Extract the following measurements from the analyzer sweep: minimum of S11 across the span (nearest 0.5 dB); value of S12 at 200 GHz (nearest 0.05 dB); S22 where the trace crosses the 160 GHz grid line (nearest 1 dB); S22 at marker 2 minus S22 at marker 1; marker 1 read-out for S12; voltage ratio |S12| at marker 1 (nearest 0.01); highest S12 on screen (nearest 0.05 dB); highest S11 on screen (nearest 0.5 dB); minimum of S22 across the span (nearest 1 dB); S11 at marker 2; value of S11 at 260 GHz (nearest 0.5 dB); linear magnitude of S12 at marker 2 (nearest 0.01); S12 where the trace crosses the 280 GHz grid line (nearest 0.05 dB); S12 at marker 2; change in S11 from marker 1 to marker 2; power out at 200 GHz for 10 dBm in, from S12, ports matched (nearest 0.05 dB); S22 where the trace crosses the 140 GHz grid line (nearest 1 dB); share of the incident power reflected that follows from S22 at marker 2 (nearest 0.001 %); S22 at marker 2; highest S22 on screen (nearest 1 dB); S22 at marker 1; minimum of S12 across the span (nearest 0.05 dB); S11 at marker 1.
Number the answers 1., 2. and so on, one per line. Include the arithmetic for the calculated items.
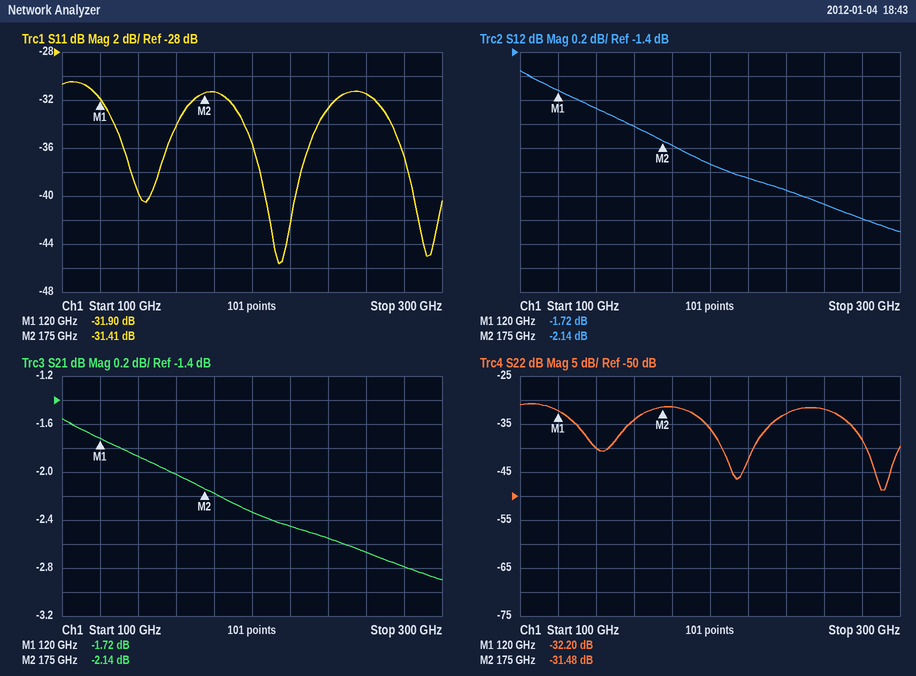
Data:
1. -45.5 dB
2. -2.35 dB
3. -34 dB
4. -31.48 − (-32.2) = 0.72 dB
5. -1.72 dB
6. 10^(-1.72/20) ≈ 0.82
7. -1.55 dB
8. -30.5 dB
9. -49 dB
10. -31.41 dB
11. -31.5 dB
12. 10^(-2.14/20) ≈ 0.78
13. -2.80 dB
14. -2.14 dB
15. -31.41 − (-31.9) = 0.49 dB
16. 10 dBm + (-2.35 dB) = 7.65 dBm
17. -40 dB
18. 10^(-31.48/10) ≈ 0.071 %
19. -31.48 dB
20. -31 dB
21. -32.20 dB
22. -2.90 dB
23. -31.90 dB
